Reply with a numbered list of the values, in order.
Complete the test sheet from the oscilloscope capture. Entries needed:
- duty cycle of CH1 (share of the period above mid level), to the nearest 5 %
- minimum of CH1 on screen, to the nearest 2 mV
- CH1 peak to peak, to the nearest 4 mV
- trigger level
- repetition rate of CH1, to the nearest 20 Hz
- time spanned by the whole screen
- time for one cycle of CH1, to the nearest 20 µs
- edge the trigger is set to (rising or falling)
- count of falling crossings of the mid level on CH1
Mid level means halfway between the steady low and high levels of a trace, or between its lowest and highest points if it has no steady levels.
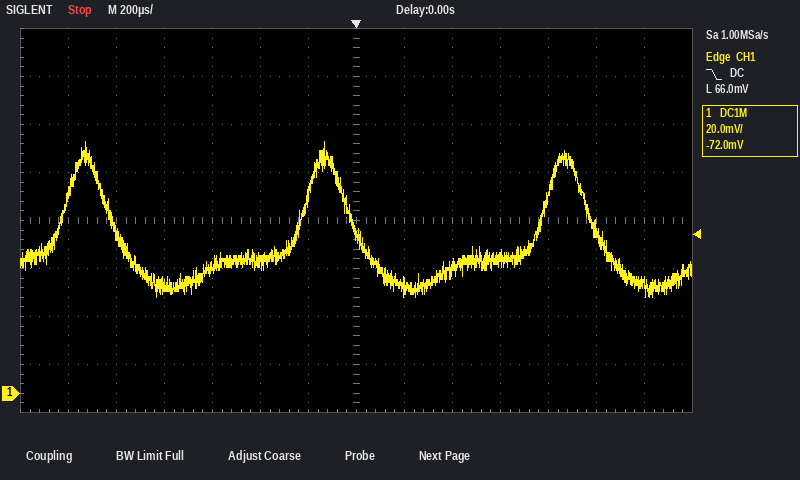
1. 20 %
2. 40 mV
3. 64 mV
4. 66.0 mV
5. 1.00 kHz
6. 2.8 ms
7. 1.00 ms
8. falling
9. 3
